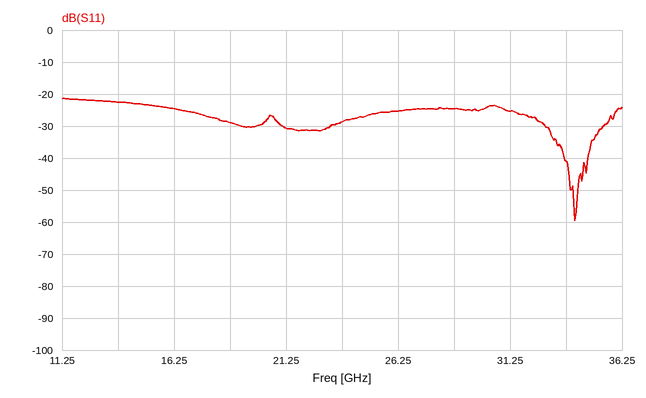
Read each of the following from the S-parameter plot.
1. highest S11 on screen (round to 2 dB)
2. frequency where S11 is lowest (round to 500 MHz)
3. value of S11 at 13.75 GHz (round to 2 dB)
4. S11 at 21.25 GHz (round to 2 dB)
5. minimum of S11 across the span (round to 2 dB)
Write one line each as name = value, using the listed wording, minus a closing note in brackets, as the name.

highest S11 on screen = -22 dB
frequency where S11 is lowest = 34.0 GHz
value of S11 at 13.75 GHz = -22 dB
S11 at 21.25 GHz = -30 dB
minimum of S11 across the span = -60 dB
